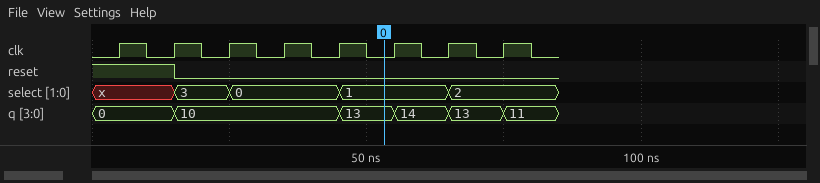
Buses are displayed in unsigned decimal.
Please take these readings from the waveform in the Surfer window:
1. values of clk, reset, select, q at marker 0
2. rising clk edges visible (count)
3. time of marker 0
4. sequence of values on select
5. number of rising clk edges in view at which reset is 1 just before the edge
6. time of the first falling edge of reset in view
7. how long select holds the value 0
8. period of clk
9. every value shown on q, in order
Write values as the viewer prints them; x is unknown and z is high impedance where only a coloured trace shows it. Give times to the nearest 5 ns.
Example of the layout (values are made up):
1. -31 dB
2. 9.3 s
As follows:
1. clk=0, reset=0, select=1, q=13
2. 8
3. 55 ns
4. x, 3, 0, 1, 2
5. 2
6. 15 ns
7. 20 ns
8. 10 ns
9. 0, 10, 13, 14, 13, 11
